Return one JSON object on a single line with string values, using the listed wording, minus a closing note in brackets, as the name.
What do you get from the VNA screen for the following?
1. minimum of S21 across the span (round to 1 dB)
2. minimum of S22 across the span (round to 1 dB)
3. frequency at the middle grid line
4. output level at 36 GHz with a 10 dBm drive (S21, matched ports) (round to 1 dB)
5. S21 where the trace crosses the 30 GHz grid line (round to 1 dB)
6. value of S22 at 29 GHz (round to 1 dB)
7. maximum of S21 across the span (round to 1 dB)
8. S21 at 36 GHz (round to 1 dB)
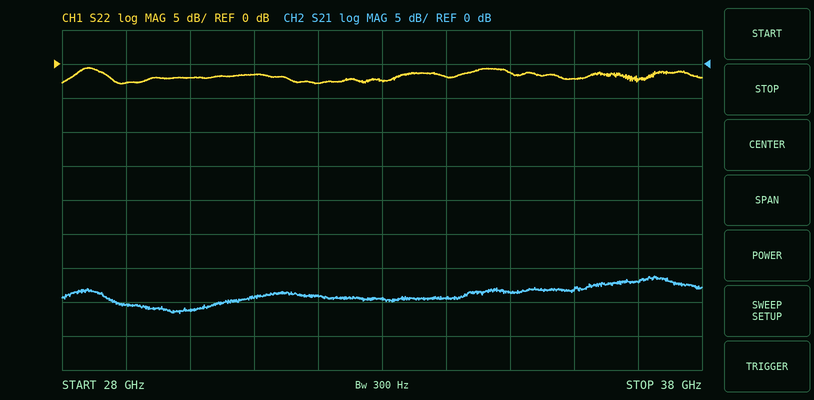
{"minimum of S21 across the span": "-37 dB", "minimum of S22 across the span": "-3 dB", "frequency at the middle grid line": "33 GHz", "output level at 36 GHz with a 10 dBm drive (S21, matched ports)": "-23 dBm", "S21 where the trace crosses the 30 GHz grid line": "-36 dB", "value of S22 at 29 GHz": "-3 dB", "maximum of S21 across the span": "-31 dB", "S21 at 36 GHz": "-33 dB"}
